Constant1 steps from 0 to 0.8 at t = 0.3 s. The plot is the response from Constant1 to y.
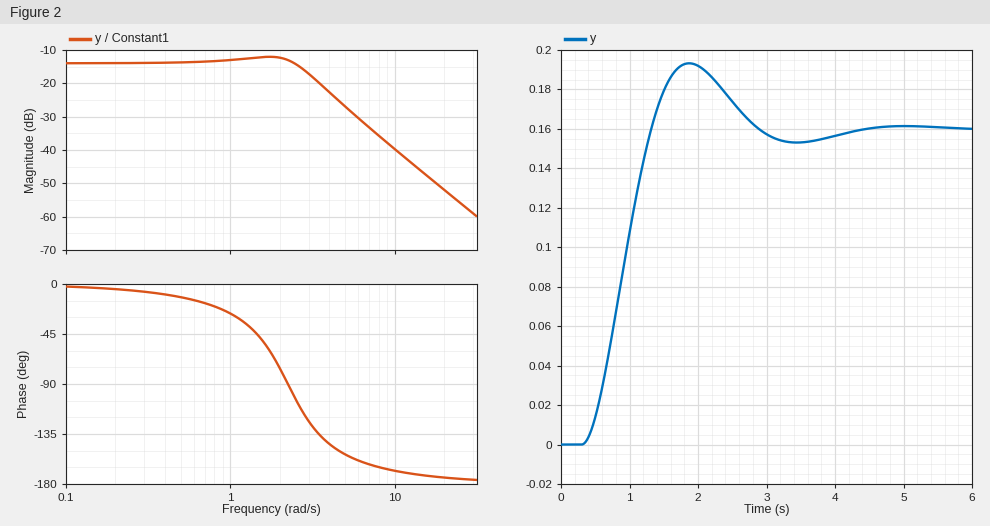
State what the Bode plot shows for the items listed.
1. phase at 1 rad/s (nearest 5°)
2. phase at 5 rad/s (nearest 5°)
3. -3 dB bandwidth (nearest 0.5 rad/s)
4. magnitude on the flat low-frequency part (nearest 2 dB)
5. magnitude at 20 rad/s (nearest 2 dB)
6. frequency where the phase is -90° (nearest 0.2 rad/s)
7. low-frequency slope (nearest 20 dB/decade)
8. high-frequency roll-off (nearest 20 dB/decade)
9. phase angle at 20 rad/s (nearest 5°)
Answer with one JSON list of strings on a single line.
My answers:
["-25°", "-155°", "3.0 rad/s", "-14 dB", "-52 dB", "2.2 rad/s", "0 dB/decade", "-40 dB/decade", "-175°"]
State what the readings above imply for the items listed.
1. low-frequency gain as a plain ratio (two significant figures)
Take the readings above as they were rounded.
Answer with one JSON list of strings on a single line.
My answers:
["0.20"]
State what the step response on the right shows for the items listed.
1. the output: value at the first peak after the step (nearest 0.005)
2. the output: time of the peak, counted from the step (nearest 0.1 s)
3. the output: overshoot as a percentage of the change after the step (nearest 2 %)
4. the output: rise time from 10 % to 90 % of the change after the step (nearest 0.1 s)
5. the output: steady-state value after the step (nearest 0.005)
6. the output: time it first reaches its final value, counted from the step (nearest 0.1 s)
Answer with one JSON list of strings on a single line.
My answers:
["0.195", "1.6 s", "20 %", "0.7 s", "0.160", "1.0 s"]
